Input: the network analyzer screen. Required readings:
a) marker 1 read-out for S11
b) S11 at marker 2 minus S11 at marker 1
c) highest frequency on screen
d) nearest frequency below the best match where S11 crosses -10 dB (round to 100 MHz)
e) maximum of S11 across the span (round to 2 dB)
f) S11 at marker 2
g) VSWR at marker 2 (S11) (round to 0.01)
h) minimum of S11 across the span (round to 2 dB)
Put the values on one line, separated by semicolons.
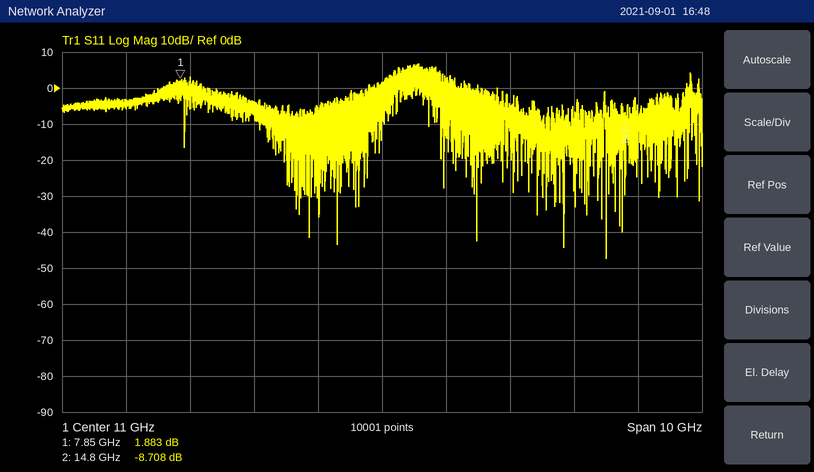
1.883 dB; -10.591 dB; 16 GHz; 14.5 GHz; 6 dB; -8.708 dB; 2.16; -48 dB
